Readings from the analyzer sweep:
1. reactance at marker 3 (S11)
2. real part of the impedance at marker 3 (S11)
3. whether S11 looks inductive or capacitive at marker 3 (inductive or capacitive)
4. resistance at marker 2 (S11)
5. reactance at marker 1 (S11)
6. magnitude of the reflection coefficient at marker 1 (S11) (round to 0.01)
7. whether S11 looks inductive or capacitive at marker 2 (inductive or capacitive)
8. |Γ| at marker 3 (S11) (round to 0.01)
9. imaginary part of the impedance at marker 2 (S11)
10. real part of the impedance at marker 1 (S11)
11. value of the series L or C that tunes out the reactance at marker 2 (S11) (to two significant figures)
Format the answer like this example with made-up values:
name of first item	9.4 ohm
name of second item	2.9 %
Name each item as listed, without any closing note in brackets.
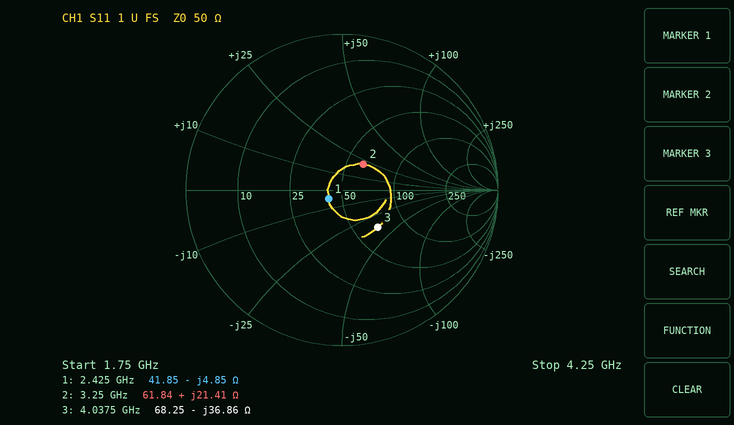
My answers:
reactance at marker 3	-36.86 Ω
real part of the impedance at marker 3	68.25 Ω
whether S11 looks inductive or capacitive at marker 3	capacitive
resistance at marker 2	61.84 Ω
reactance at marker 1	-4.85 Ω
magnitude of the reflection coefficient at marker 1 (S11)	0.10
whether S11 looks inductive or capacitive at marker 2	inductive
|Γ| at marker 3 (S11)	0.33
imaginary part of the impedance at marker 2	+21.41 Ω
real part of the impedance at marker 1	41.85 Ω
value of the series L or C that tunes out the reactance at marker 2 (S11)	2.3 pF
